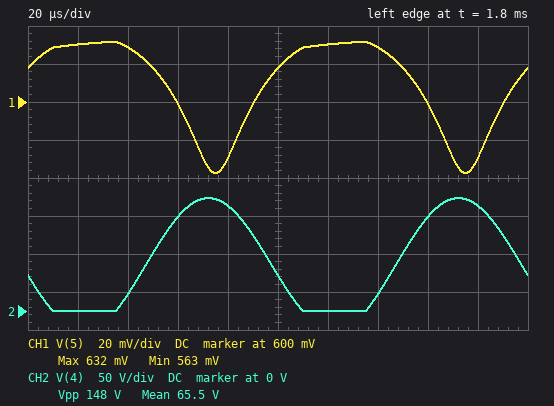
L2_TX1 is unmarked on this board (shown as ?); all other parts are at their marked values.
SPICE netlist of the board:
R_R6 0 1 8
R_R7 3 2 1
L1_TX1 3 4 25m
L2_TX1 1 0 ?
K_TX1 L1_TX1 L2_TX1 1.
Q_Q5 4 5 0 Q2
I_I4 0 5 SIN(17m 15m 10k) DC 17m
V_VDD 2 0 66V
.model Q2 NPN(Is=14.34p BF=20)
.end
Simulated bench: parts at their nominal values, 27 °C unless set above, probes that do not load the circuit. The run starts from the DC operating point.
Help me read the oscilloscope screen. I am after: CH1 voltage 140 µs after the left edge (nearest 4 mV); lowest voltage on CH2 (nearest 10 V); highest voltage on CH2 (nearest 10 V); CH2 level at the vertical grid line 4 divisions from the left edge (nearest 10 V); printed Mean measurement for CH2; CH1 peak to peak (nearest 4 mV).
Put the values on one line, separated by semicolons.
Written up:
628 mV; 0 V; 150 V; 140 V; 65.5 V; 68 mV
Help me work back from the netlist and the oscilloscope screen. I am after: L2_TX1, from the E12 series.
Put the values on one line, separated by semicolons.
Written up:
680 µH
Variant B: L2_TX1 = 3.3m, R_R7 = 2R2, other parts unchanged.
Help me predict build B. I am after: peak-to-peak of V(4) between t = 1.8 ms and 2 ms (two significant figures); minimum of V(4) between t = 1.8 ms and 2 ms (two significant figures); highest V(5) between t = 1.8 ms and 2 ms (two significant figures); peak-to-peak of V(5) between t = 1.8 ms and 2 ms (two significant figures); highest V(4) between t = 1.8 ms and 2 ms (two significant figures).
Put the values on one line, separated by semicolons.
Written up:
38 V; 46 V; 630 mV; 72 mV; 84 V
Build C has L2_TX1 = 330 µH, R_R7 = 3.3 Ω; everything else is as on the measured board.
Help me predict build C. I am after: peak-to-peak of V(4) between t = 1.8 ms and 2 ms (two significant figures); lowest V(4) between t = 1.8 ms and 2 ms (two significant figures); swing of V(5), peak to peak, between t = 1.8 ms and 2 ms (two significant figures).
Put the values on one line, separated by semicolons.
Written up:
190 V; 90 mV; 61 mV
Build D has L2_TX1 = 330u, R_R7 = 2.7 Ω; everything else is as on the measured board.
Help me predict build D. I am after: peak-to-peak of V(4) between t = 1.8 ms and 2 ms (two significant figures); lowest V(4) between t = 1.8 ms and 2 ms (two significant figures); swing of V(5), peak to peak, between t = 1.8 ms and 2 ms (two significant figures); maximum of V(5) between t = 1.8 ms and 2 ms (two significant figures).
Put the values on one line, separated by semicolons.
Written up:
190 V; 90 mV; 61 mV; 620 mV
